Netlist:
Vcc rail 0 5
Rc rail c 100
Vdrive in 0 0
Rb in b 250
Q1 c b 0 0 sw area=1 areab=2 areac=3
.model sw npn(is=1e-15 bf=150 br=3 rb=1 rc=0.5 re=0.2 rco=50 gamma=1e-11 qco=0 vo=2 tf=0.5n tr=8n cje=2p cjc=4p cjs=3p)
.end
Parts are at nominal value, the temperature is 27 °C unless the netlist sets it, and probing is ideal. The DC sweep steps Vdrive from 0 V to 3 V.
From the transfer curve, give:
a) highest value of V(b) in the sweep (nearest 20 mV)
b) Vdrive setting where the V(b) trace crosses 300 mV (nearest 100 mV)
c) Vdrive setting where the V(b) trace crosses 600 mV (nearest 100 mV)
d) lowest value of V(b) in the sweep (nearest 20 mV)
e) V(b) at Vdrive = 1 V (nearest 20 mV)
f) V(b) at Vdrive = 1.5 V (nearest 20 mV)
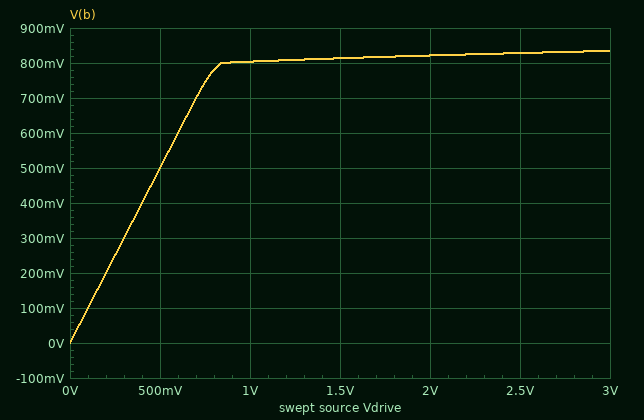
840 mV
300 mV
600 mV
0 V
800 mV
820 mV
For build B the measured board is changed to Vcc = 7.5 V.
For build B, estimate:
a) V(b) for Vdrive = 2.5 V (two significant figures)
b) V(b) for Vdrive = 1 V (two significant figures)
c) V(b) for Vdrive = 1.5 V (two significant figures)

830 mV
810 mV
820 mV
